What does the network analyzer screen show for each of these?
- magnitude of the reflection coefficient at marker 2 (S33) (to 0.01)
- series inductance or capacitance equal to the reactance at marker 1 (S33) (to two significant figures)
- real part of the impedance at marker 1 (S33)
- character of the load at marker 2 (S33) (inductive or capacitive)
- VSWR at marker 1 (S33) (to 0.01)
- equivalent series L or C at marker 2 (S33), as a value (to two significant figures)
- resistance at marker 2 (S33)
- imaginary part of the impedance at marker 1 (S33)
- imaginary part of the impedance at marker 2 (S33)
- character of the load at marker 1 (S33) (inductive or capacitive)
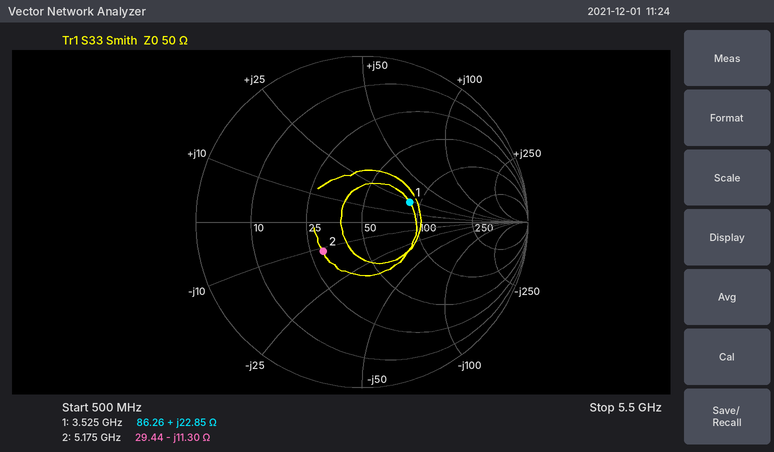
0.29
1.0 nH
86.26 Ω
capacitive
1.90
2.7 pF
29.44 Ω
+22.85 Ω
-11.30 Ω
inductive
